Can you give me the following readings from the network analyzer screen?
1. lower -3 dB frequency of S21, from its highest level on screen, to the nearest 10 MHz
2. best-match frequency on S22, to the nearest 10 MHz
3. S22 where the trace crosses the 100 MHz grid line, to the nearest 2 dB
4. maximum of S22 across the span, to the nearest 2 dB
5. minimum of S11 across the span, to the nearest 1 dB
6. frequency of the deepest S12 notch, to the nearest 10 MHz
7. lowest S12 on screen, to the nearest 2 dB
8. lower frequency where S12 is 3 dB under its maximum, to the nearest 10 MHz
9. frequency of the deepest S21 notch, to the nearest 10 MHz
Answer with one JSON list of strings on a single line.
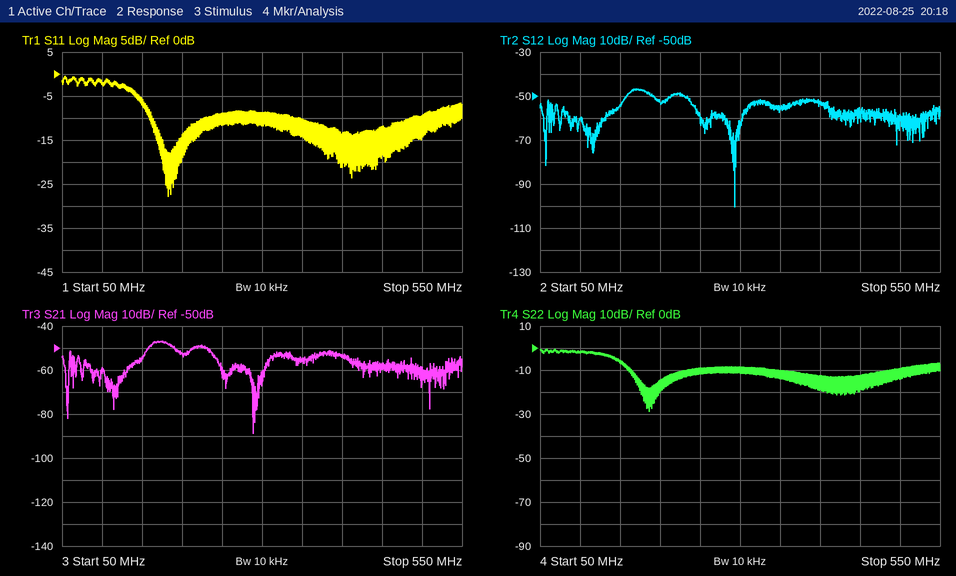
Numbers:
["160 MHz", "190 MHz", "-2 dB", "0 dB", "-28 dB", "290 MHz", "-100 dB", "160 MHz", "290 MHz"]
